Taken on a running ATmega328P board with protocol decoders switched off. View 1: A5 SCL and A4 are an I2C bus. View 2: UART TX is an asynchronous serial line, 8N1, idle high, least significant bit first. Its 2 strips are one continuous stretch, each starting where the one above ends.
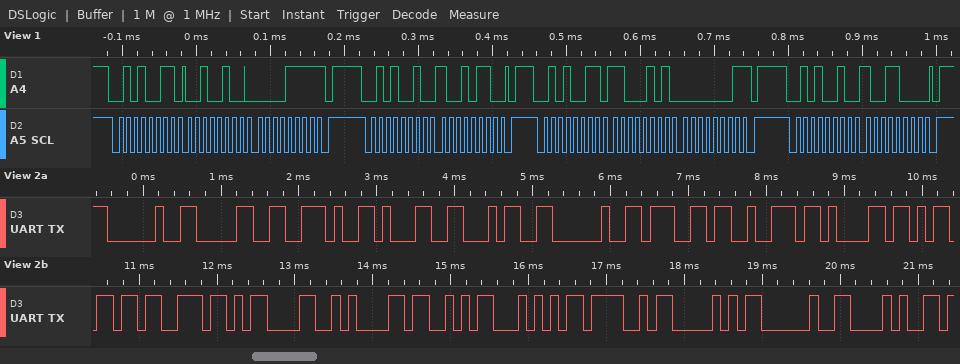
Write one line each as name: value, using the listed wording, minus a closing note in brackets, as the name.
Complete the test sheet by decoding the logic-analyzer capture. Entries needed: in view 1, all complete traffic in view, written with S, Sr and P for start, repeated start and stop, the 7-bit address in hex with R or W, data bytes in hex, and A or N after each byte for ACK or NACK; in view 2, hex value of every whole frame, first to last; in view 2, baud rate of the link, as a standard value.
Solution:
in view 1, all complete traffic in view, written with S, Sr and P for start, repeated start and stop, the 7-bit address in hex with R or W, data bytes in hex, and A or N after each byte for ACK or NACK: S 29R A 24 A 0F N P S 29W A 96 A P S 29R A C5 A 01 N P S 29W A 98 A P
in view 2, hex value of every whole frame, first to last: 20 30 2E 31 34 20 67 72 61 6D 73 0D 0A 53 54 4F 50 20 28
in view 2, baud rate of the link, as a standard value: 9600 baud
